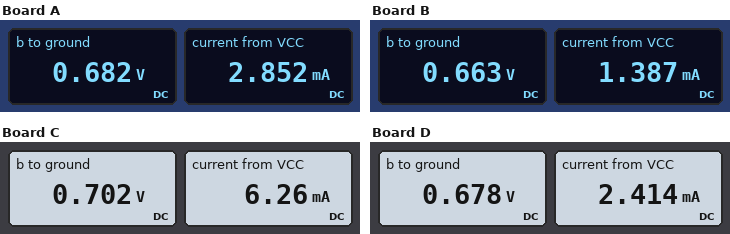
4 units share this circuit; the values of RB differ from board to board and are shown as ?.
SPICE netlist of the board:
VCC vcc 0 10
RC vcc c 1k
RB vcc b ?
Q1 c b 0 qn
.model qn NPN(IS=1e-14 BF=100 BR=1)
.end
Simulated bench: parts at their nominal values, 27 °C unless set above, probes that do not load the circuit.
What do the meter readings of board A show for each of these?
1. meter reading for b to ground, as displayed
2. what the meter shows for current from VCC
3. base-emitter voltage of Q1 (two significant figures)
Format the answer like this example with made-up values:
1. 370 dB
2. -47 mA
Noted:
1. 0.682 V
2. 2.852 mA
3. 680 mV
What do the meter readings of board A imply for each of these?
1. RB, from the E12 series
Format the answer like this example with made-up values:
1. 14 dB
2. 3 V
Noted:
1. 330 kΩ
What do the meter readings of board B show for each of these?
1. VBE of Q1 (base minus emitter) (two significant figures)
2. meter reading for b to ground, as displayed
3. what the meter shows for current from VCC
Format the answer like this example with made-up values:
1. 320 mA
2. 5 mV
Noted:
1. 660 mV
2. 0.663 V
3. 1.387 mA
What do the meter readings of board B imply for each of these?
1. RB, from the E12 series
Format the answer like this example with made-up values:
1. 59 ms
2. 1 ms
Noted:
1. 680 kΩ
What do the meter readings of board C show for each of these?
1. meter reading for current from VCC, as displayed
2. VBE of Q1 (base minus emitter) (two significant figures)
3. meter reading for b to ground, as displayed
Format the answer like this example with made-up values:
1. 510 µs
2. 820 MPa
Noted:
1. 6.26 mA
2. 700 mV
3. 0.702 V
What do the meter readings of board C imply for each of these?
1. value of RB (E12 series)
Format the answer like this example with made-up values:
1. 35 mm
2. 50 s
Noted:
1. 150 kΩ
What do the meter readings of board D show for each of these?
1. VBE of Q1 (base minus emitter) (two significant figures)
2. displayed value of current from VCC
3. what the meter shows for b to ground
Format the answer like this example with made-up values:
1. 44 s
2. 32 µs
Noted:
1. 680 mV
2. 2.414 mA
3. 0.678 V
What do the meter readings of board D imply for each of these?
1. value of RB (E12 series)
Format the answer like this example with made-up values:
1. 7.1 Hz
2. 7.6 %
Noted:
1. 390 kΩ
